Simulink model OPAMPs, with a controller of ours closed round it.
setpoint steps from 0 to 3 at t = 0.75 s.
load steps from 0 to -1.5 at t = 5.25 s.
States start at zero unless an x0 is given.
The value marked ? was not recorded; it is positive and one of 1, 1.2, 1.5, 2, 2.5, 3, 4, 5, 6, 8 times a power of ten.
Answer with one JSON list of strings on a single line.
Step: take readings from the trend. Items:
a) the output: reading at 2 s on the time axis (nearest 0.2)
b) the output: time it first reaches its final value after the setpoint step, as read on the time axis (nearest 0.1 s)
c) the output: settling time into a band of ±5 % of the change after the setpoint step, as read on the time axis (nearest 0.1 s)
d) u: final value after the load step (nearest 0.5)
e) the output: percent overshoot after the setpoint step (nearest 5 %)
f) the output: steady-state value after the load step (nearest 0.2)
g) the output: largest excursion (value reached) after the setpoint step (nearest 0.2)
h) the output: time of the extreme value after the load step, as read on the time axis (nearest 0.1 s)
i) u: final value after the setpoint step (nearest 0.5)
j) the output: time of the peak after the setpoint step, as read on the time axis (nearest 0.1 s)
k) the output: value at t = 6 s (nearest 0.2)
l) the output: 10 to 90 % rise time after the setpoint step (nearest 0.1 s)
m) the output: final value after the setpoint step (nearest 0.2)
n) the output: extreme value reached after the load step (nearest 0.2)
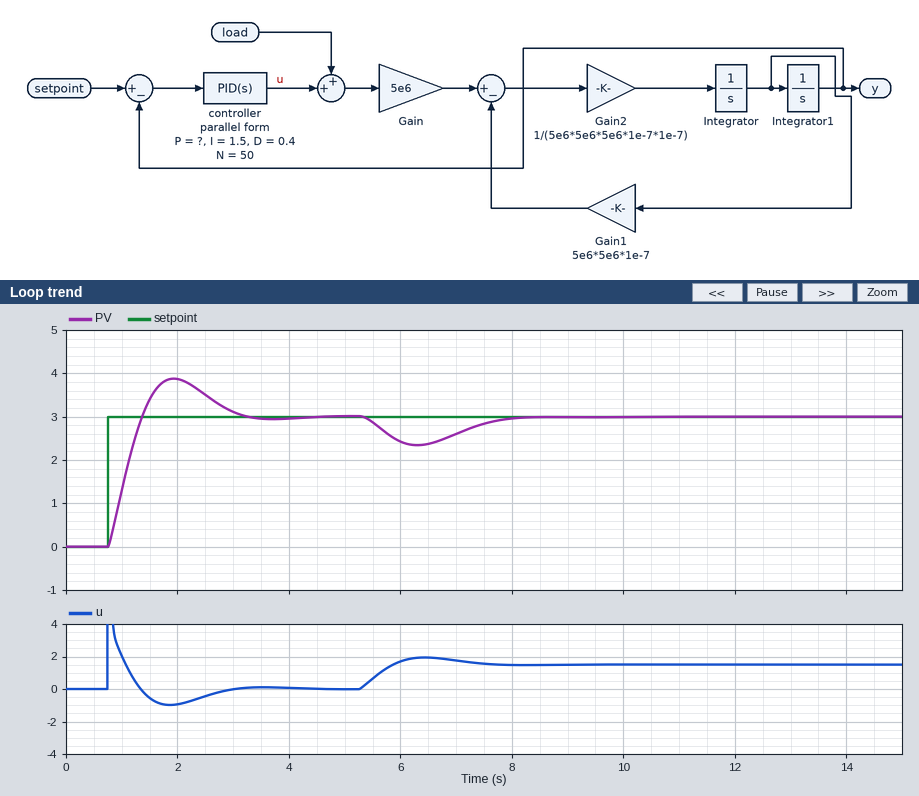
["3.8", "1.4 s", "2.9 s", "1.5", "30 %", "3.0", "3.8", "6.3 s", "0.0", "1.9 s", "2.4", "0.5 s", "3.0", "2.4"]
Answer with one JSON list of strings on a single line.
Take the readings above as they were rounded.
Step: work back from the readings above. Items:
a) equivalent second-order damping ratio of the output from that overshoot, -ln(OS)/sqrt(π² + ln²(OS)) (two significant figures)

["0.36"]
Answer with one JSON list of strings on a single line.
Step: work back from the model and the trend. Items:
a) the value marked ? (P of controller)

["2"]
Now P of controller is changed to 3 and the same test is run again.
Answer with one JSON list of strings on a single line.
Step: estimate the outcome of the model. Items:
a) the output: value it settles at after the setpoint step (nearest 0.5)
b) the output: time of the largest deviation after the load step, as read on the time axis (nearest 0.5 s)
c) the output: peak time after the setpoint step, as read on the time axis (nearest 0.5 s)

["3.0", "6.0 s", "1.5 s"]
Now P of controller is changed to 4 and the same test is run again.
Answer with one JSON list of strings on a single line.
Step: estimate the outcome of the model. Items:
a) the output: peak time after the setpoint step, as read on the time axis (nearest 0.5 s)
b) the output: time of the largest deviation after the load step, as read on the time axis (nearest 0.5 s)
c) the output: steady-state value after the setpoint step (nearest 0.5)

["1.5 s", "6.0 s", "3.0"]
